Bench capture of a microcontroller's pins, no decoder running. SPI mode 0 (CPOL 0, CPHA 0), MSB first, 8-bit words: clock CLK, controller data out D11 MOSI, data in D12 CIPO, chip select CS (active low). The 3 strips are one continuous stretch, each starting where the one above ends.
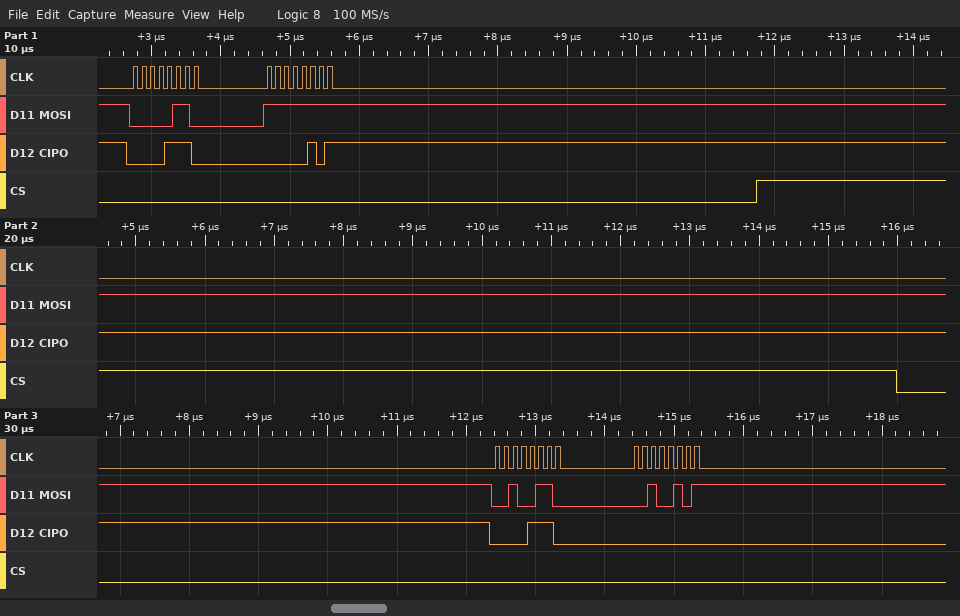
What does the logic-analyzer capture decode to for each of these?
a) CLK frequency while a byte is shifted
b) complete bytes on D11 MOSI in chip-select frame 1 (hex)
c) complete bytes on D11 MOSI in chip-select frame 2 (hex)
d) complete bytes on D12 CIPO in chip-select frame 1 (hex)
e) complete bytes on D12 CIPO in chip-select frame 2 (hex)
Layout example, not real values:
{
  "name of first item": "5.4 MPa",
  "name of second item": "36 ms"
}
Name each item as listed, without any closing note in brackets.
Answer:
{
  "CLK frequency while a byte is shifted": "8 MHz",
  "complete bytes on D11 MOSI in chip-select frame 1": "06 FF",
  "complete bytes on D11 MOSI in chip-select frame 2": "26 25",
  "complete bytes on D12 CIPO in chip-select frame 1": "0E 05",
  "complete bytes on D12 CIPO in chip-select frame 2": "0E 00"
}
